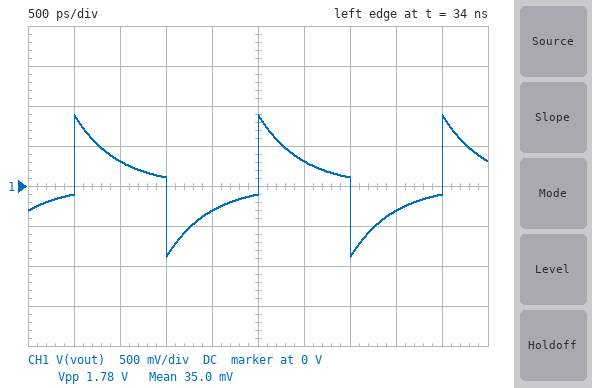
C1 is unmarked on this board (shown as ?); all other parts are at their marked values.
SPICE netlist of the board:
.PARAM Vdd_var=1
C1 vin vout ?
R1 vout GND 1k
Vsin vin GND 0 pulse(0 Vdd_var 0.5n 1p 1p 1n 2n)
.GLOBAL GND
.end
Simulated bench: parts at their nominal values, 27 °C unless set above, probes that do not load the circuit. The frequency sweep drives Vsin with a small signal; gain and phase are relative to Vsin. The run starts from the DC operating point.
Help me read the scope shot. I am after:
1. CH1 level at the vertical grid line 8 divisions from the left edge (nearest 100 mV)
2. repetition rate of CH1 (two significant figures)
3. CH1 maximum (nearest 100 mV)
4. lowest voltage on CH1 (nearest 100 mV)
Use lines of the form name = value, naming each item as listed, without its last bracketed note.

CH1 level at the vertical grid line 8 divisions from the left edge = -300 mV
repetition rate of CH1 = 500 MHz
CH1 maximum = 900 mV
lowest voltage on CH1 = -900 mV
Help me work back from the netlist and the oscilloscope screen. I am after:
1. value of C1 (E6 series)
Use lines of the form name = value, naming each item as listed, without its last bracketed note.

value of C1 = 470 fF
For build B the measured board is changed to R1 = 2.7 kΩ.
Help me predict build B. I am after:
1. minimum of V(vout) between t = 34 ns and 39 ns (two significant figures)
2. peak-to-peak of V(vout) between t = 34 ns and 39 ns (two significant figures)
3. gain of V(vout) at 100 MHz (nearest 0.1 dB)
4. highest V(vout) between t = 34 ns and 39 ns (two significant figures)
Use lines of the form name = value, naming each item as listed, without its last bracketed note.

minimum of V(vout) between t = 34 ns and 39 ns = -690 mV
peak-to-peak of V(vout) between t = 34 ns and 39 ns = 1.4 V
gain of V(vout) at 100 MHz = -4.1 dB
highest V(vout) between t = 34 ns and 39 ns = 690 mV
